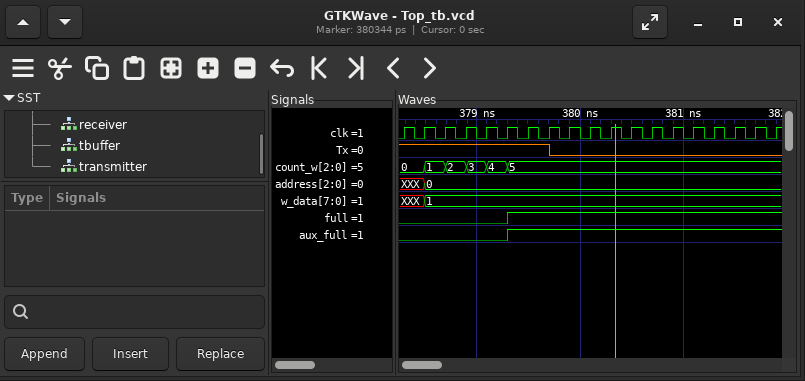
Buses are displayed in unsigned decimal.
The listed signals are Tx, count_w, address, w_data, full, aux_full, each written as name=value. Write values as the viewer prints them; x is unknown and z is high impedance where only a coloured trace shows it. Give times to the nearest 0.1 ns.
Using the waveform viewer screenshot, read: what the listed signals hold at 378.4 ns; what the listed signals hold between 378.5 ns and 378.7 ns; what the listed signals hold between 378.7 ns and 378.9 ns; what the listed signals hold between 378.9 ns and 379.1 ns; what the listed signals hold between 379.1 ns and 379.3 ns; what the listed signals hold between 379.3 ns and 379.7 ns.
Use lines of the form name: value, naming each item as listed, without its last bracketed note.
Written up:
what the listed signals hold at 378.4 ns: Tx=1, count_w=0, address=XXX, w_data=XXX, full=0, aux_full=0
what the listed signals hold between 378.5 ns and 378.7 ns: Tx=1, count_w=1, address=0, w_data=1, full=0, aux_full=0
what the listed signals hold between 378.7 ns and 378.9 ns: Tx=1, count_w=2, address=0, w_data=1, full=0, aux_full=0
what the listed signals hold between 378.9 ns and 379.1 ns: Tx=1, count_w=3, address=0, w_data=1, full=0, aux_full=0
what the listed signals hold between 379.1 ns and 379.3 ns: Tx=1, count_w=4, address=0, w_data=1, full=0, aux_full=0
what the listed signals hold between 379.3 ns and 379.7 ns: Tx=1, count_w=5, address=0, w_data=1, full=1, aux_full=1
